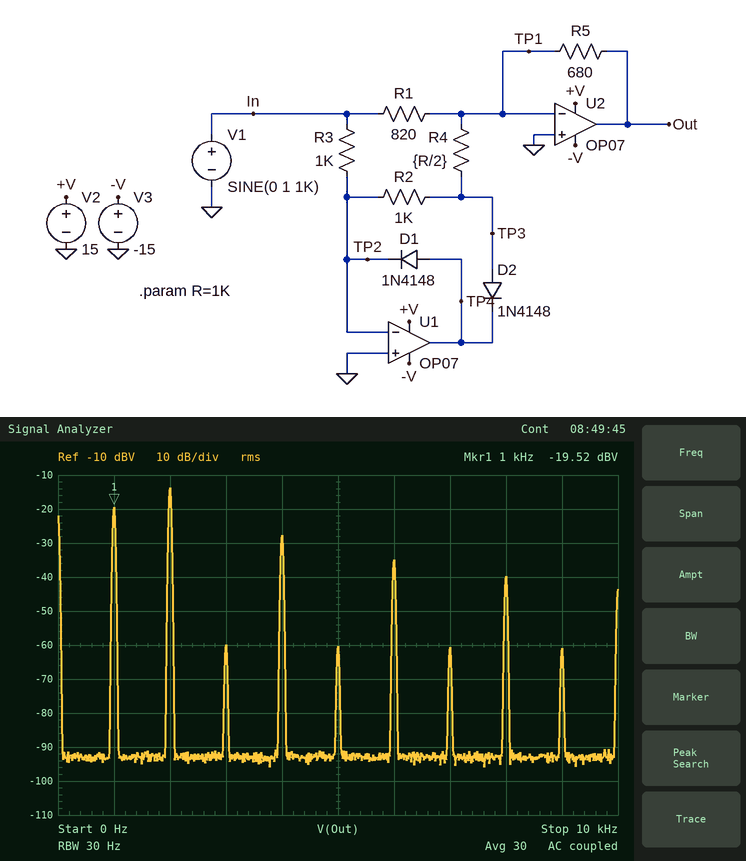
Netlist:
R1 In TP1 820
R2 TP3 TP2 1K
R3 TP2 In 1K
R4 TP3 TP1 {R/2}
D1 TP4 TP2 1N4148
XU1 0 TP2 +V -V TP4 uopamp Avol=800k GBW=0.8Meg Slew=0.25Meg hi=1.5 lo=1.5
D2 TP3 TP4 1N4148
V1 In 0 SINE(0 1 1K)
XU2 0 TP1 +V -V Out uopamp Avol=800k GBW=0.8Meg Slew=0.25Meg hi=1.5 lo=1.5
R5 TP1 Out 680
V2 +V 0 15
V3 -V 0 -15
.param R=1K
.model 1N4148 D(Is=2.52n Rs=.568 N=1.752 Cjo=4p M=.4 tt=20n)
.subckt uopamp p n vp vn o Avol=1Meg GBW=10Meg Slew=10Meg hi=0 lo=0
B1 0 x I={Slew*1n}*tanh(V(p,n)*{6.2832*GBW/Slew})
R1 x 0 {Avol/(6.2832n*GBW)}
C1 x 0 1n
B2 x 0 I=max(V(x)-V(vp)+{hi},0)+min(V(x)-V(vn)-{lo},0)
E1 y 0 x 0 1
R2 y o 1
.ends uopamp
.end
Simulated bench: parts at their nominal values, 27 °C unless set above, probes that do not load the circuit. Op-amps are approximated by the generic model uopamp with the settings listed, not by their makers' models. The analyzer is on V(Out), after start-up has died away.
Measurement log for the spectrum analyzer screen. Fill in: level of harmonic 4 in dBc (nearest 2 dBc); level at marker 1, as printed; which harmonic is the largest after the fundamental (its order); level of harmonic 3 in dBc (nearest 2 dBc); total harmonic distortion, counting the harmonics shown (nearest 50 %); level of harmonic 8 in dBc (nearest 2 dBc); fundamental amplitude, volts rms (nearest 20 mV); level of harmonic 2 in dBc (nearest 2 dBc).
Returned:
-8 dBc
-19.52 dBV
2
-40 dBc
200 %
-20 dBc
100 mV
6 dBc
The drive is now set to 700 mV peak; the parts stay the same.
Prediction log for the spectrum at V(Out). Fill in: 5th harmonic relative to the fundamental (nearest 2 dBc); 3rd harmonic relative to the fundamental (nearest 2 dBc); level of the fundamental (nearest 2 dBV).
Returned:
-38 dBc
-38 dBc
-22 dBV
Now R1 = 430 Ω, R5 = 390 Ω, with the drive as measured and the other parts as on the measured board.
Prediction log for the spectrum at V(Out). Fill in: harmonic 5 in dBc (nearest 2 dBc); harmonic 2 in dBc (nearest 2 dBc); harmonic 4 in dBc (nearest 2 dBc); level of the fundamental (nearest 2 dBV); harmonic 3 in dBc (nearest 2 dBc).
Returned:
-56 dBc
-10 dBc
-24 dBc
-8 dBV
-56 dBc
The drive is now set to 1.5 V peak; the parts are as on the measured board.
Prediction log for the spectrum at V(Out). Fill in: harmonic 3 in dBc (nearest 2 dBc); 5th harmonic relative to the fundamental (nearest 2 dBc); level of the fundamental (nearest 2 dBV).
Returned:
-44 dBc
-44 dBc
-16 dBV
